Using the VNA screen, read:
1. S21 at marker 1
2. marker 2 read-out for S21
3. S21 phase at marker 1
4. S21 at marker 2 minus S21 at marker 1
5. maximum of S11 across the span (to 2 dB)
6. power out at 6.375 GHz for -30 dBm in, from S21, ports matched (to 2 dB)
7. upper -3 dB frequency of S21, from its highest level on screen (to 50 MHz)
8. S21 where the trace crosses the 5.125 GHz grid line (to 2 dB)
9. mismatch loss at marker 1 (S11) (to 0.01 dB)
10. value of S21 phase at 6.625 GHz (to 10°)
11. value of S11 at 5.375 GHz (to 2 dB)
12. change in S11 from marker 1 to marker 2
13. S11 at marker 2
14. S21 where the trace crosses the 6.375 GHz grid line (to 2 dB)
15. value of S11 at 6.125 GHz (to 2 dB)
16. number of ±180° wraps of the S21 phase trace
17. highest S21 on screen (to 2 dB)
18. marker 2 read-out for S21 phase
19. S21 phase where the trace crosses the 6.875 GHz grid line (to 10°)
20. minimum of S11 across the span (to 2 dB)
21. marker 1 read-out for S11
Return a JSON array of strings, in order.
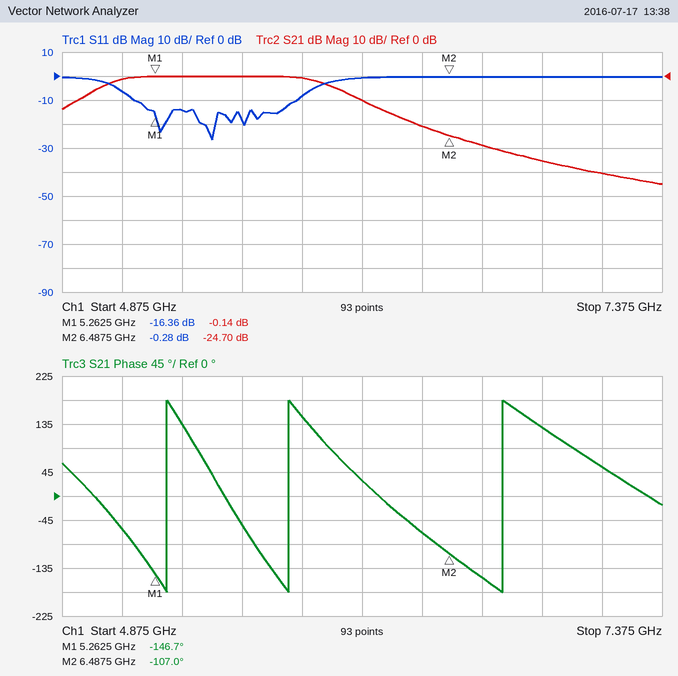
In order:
["-0.14 dB", "-24.70 dB", "-146.7°", "-24.56 dB", "0 dB", "-50 dBm", "5.95 GHz", "-2 dB", "0.10 dB", "-150°", "-14 dB", "16.08 dB", "-0.28 dB", "-20 dB", "0 dB", "3", "0 dB", "-107.0°", "130°", "-26 dB", "-16.36 dB"]
